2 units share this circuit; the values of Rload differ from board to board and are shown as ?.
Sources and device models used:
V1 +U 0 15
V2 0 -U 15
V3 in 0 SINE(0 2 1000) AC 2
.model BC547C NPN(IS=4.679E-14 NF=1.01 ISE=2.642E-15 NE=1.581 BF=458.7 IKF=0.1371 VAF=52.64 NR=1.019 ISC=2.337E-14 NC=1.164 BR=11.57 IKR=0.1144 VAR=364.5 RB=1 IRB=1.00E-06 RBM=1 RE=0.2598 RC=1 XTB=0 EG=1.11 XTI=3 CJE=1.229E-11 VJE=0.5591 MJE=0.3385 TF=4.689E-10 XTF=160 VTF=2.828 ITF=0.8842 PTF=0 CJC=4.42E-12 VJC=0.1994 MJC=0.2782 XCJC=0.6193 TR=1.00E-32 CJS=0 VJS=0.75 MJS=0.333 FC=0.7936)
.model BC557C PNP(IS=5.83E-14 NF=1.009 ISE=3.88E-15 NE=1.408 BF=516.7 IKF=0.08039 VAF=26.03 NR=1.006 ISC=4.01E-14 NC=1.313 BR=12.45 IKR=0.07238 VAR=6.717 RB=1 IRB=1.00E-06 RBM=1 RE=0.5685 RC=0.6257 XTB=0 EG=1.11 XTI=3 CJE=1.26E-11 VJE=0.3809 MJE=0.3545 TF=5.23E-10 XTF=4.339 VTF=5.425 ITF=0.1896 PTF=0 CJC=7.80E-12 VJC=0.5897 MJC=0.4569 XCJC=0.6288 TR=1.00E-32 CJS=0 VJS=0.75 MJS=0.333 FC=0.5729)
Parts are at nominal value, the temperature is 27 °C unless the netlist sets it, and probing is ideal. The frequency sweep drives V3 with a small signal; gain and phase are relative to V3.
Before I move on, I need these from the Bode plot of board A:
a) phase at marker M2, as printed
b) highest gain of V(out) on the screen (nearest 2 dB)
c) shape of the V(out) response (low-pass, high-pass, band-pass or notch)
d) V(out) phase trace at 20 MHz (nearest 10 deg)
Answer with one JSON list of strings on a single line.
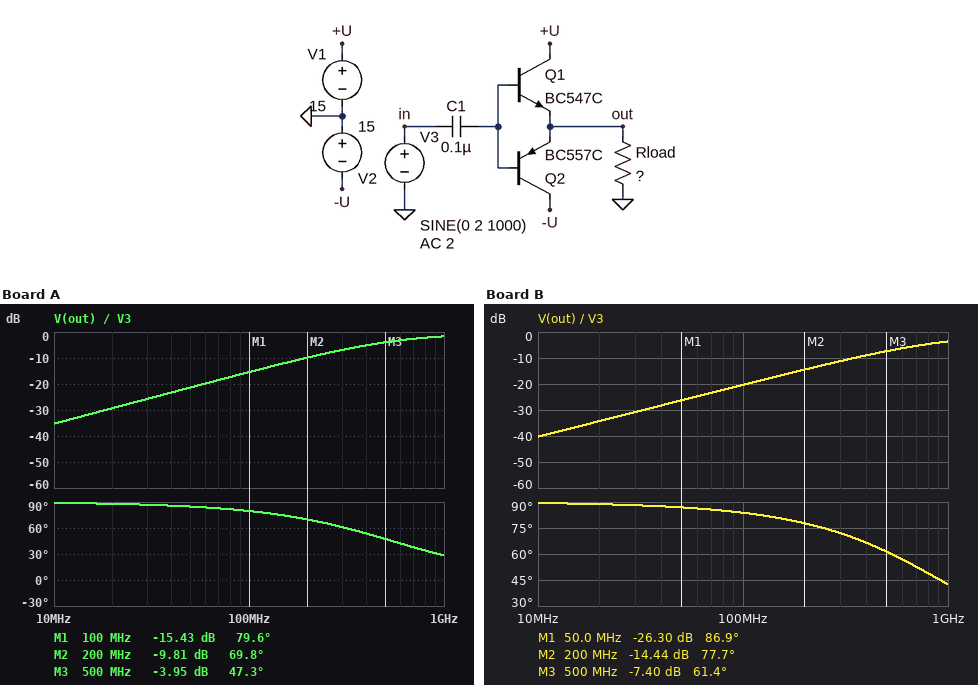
["69.8 deg", "-2 dB", "high-pass", "90 deg"]
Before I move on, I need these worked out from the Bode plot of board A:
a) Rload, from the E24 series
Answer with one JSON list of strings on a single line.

["11 Ω"]
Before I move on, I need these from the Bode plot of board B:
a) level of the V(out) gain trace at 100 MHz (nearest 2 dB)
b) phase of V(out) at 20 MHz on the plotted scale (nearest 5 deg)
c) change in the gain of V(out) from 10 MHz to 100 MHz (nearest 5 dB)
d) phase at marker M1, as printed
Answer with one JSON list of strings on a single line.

["-20 dB", "90 deg", "20 dB", "86.9 deg"]
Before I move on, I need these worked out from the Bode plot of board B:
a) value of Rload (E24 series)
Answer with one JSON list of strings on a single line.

["6.2 Ω"]
